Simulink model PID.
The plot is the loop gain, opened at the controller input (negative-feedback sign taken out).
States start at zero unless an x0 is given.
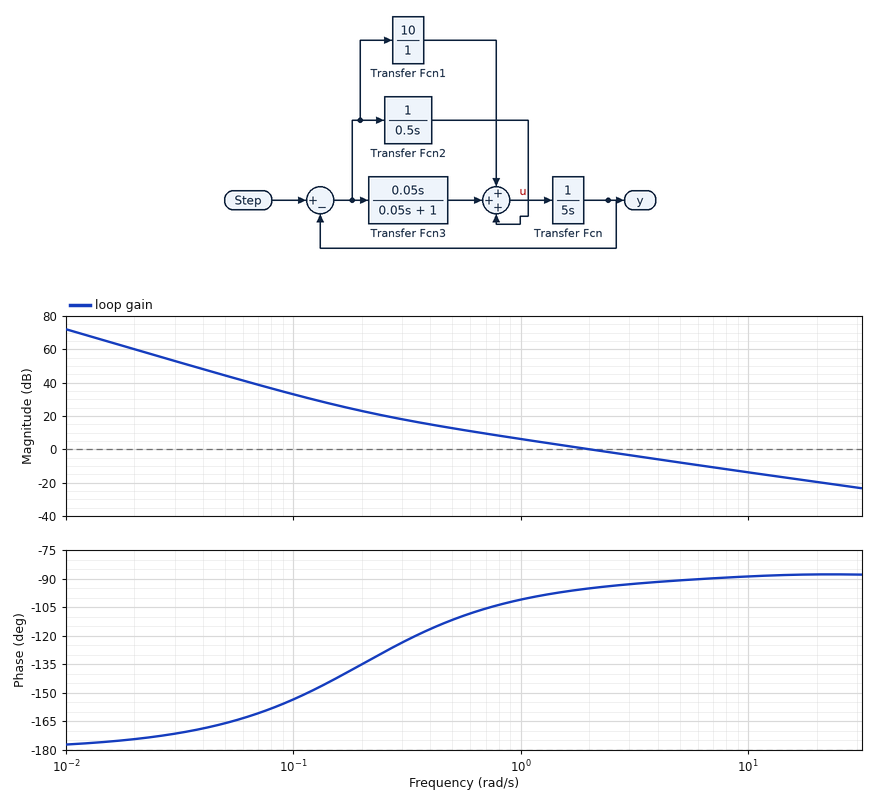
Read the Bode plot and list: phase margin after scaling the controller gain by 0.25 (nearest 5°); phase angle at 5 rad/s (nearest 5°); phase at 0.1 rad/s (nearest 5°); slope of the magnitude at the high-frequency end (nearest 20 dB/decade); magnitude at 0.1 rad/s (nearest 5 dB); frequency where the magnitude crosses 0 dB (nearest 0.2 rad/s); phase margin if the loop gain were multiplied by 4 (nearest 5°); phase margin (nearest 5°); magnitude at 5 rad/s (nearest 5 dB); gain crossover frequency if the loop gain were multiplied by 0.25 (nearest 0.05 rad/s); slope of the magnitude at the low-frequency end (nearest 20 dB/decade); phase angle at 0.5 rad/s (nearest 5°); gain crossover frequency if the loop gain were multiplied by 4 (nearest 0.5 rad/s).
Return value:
70°
-90°
-155°
-20 dB/decade
35 dB
2.0 rad/s
90°
85°
-10 dB
0.55 rad/s
-40 dB/decade
-110°
8.0 rad/s
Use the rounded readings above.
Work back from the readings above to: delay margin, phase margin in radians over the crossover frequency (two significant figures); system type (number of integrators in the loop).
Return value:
0.74 s
2
